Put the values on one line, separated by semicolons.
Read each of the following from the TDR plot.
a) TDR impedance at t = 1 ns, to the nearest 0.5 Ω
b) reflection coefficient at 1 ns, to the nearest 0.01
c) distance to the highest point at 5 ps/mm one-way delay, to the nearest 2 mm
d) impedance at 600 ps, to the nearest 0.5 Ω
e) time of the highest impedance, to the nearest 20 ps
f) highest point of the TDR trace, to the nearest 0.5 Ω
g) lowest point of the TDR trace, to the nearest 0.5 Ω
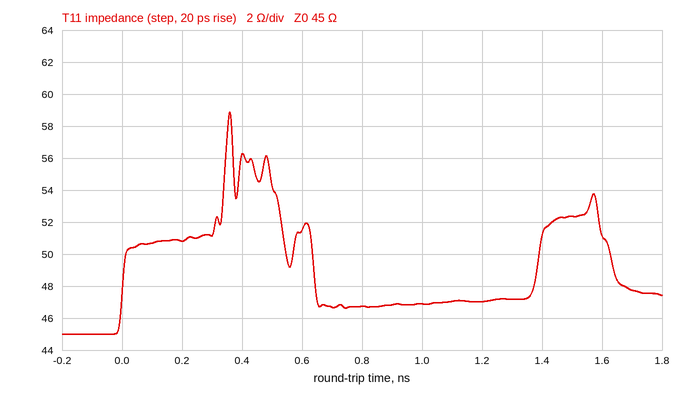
47.0 Ω; +0.02; 36 mm; 51.5 Ω; 360 ps; 59.0 Ω; 45.0 Ω
